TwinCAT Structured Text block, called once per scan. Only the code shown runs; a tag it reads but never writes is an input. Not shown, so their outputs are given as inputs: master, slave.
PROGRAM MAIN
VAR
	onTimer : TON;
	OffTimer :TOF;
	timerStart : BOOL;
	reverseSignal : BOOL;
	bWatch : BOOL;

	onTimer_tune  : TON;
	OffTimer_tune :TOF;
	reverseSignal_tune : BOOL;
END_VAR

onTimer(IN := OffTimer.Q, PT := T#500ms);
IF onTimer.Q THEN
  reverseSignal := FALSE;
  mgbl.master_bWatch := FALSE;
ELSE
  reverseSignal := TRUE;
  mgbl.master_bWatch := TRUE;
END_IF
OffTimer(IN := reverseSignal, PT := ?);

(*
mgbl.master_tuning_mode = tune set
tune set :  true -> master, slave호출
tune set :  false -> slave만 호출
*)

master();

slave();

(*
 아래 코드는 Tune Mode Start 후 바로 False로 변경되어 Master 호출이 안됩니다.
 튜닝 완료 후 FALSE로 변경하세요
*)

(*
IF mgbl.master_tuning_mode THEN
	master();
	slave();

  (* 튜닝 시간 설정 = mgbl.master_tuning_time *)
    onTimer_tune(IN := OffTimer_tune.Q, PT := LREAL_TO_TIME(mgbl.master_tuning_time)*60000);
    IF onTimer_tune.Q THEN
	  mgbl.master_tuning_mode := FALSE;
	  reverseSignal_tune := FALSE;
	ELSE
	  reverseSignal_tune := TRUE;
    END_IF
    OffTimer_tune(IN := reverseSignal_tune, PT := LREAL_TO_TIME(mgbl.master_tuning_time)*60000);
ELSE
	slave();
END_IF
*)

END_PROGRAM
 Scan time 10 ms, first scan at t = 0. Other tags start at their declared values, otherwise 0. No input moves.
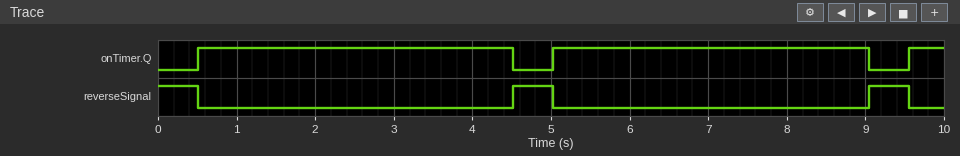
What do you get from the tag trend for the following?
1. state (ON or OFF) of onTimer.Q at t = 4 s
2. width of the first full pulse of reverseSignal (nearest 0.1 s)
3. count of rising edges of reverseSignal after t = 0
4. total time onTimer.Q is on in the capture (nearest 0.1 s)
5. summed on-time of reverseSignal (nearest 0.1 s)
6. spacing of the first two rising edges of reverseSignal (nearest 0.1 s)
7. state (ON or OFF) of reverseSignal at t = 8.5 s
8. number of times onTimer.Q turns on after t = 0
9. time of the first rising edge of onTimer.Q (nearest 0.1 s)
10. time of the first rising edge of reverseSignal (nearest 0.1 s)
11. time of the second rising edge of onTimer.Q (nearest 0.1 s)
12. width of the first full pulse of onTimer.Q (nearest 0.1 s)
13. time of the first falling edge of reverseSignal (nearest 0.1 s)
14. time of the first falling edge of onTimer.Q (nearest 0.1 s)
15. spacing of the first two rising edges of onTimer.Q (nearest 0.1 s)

ON
0.5 s
2
8.5 s
1.5 s
4.5 s
OFF
3
0.5 s
4.5 s
5.0 s
4.0 s
0.5 s
4.5 s
4.5 s
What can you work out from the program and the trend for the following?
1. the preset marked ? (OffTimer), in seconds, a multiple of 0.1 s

4.0 s
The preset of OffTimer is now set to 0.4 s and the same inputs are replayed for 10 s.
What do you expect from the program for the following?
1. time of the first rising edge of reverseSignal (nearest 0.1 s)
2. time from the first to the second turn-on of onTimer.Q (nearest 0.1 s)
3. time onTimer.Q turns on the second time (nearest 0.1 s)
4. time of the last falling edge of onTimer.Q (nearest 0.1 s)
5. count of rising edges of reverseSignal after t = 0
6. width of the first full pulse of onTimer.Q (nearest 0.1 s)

0.9 s
0.9 s
1.4 s
9.2 s
10
0.4 s
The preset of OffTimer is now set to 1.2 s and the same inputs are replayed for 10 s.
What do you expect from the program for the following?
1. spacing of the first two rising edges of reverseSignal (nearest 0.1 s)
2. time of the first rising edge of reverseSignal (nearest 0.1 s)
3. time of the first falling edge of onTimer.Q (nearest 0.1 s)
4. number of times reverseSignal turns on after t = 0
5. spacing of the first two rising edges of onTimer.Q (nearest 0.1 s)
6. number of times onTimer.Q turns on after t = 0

1.7 s
1.7 s
1.7 s
5
1.7 s
6
